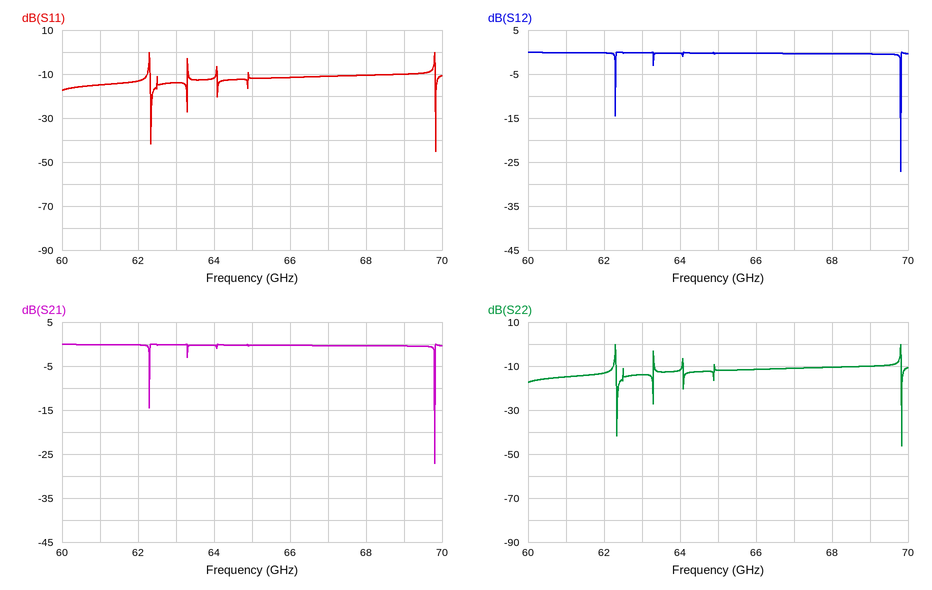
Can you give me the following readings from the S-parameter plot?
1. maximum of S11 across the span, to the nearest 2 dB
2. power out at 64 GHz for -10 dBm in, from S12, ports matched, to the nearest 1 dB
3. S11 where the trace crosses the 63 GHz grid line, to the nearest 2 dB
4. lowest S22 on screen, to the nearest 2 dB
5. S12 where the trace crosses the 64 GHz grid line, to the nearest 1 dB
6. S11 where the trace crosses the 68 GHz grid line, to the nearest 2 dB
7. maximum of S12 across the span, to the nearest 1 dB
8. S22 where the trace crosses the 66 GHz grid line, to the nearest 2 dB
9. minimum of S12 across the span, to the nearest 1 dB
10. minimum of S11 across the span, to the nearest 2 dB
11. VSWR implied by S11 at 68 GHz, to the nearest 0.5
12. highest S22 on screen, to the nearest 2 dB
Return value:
0 dB
-10 dBm
-14 dB
-46 dB
0 dB
-10 dB
0 dB
-12 dB
-27 dB
-46 dB
2.0
0 dB
